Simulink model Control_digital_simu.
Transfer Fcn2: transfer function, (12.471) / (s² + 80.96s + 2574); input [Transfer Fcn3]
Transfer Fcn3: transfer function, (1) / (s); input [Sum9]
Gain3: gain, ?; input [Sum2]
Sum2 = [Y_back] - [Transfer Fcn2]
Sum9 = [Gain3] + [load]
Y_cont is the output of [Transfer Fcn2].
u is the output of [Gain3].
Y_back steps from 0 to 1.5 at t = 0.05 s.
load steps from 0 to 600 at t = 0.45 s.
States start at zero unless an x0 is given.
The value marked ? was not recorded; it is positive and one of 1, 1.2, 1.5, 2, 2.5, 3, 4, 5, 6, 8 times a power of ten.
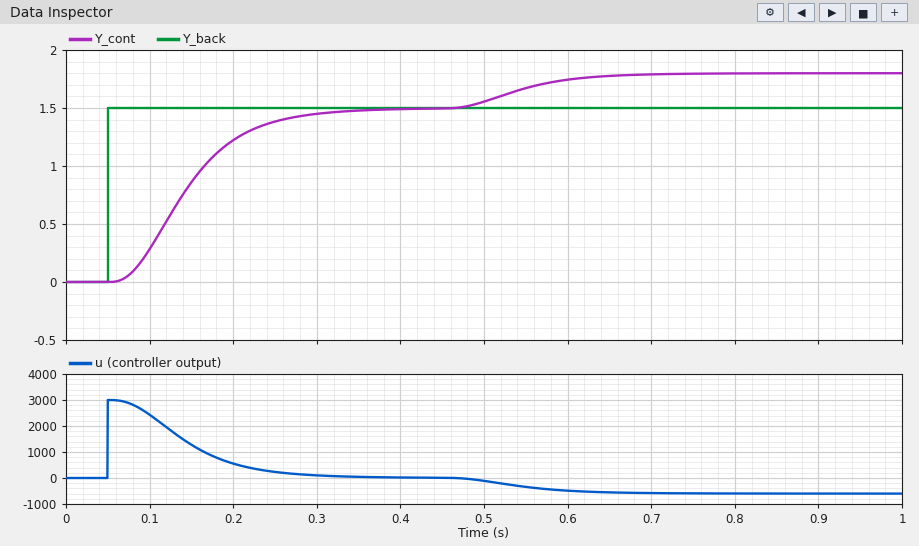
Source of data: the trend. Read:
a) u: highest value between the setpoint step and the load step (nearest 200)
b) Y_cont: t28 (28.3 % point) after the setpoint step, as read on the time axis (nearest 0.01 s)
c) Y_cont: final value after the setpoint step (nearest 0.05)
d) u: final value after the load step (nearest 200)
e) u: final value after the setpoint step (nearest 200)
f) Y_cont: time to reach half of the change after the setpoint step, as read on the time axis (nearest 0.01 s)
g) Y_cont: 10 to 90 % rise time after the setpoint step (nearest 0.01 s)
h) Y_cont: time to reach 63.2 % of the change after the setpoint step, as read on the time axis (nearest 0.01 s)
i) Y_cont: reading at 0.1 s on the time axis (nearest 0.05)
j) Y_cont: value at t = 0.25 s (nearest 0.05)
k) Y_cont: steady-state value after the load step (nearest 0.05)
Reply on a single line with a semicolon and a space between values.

3000; 0.11 s; 1.50; -600; 0; 0.14 s; 0.15 s; 0.16 s; 0.30; 1.40; 1.80
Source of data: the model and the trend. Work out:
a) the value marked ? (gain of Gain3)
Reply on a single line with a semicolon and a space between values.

2000
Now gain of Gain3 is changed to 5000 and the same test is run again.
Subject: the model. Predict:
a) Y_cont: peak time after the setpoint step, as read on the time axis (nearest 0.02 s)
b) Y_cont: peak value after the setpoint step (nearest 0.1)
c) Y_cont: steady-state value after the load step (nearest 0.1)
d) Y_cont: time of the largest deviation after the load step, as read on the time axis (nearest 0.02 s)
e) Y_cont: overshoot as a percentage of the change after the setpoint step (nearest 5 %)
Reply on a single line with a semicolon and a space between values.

0.18 s; 1.8; 1.6; 0.58 s; 20 %
